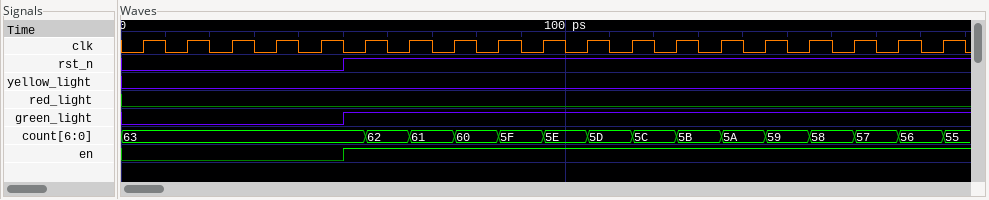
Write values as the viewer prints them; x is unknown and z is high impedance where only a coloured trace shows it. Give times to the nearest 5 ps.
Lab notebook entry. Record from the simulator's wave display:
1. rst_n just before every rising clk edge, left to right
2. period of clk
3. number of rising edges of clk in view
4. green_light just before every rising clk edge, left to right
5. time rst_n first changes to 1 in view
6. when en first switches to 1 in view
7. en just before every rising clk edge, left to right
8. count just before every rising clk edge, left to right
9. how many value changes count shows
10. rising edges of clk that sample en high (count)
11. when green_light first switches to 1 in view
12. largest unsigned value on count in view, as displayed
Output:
0 0 0 0 0 1 1 1 1 1 1 1 1 1 1 1 1 1 1
10 ps
19
0 0 0 0 0 1 1 1 1 1 1 1 1 1 1 1 1 1 1
50 ps
50 ps
0 0 0 0 0 1 1 1 1 1 1 1 1 1 1 1 1 1 1
63, 63, 63, 63, 63, 63, 62, 61, 60, 5F, 5E, 5D, 5C, 5B, 5A, 59, 58, 57, 56
14
14
50 ps
63
